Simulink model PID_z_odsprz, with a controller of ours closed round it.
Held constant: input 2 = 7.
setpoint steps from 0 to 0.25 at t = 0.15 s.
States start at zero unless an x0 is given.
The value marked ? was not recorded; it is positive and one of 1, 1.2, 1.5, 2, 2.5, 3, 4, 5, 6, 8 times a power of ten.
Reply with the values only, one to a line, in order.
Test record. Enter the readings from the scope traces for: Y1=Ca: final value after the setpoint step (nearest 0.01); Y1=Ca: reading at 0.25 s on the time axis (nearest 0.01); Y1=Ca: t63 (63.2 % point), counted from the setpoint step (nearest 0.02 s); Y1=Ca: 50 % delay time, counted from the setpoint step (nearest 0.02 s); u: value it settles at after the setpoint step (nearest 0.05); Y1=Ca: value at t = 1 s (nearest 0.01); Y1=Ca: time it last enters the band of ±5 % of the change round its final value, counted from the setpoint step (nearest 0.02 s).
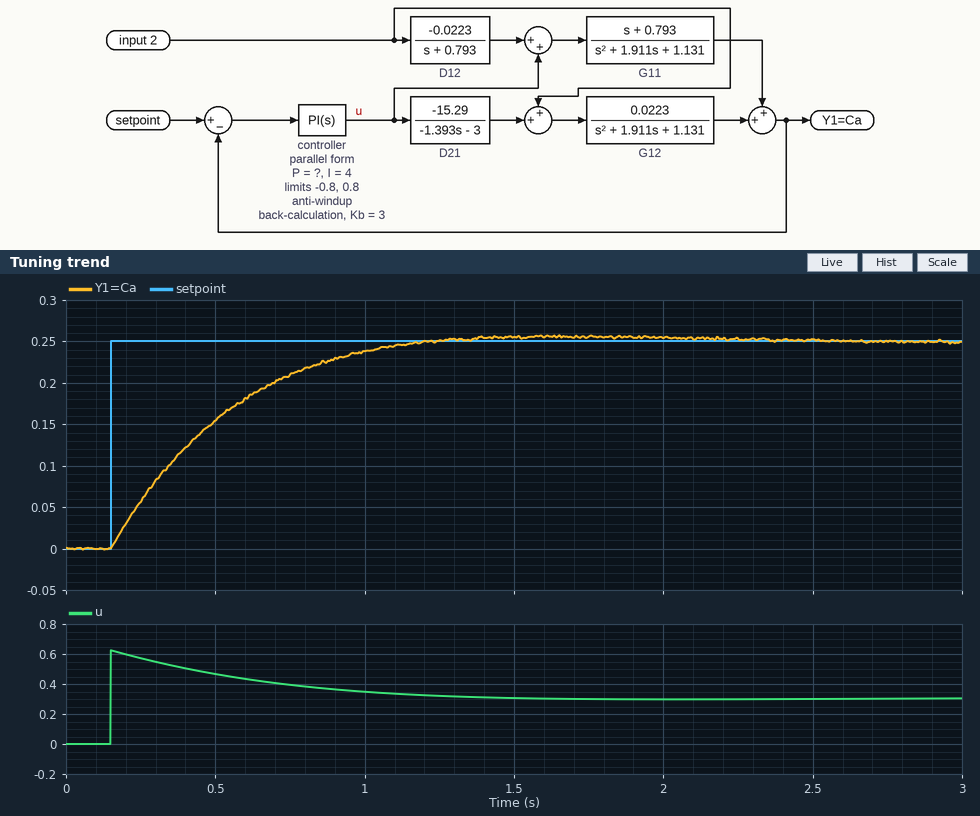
0.25
0.06
0.36 s
0.26 s
0.30
0.24
0.84 s
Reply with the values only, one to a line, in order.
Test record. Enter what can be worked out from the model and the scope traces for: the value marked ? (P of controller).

2.5
